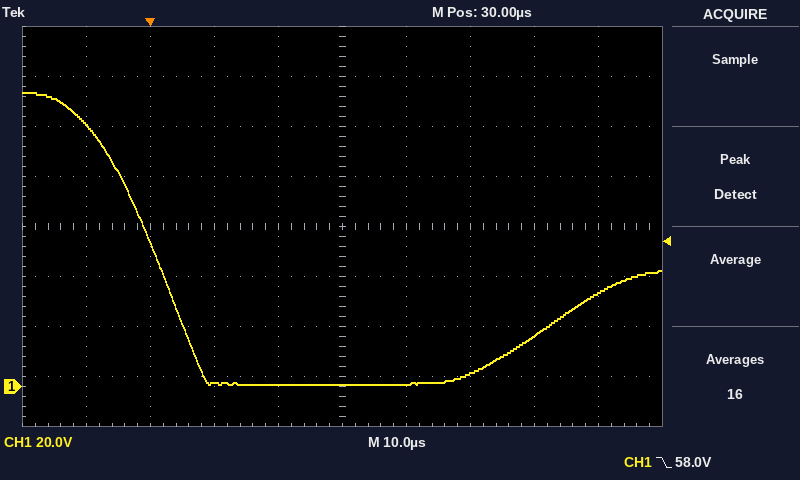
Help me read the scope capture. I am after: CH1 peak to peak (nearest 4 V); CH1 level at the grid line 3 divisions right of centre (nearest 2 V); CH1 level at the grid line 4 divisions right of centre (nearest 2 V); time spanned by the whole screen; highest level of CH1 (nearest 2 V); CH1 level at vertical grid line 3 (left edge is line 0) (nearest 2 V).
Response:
116 V
20 V
38 V
100 µs
118 V
2 V
